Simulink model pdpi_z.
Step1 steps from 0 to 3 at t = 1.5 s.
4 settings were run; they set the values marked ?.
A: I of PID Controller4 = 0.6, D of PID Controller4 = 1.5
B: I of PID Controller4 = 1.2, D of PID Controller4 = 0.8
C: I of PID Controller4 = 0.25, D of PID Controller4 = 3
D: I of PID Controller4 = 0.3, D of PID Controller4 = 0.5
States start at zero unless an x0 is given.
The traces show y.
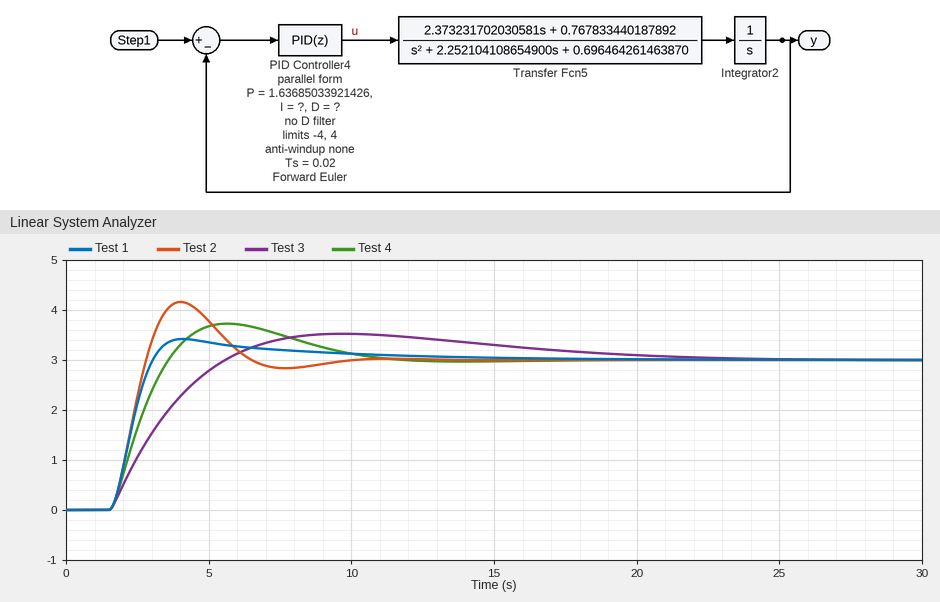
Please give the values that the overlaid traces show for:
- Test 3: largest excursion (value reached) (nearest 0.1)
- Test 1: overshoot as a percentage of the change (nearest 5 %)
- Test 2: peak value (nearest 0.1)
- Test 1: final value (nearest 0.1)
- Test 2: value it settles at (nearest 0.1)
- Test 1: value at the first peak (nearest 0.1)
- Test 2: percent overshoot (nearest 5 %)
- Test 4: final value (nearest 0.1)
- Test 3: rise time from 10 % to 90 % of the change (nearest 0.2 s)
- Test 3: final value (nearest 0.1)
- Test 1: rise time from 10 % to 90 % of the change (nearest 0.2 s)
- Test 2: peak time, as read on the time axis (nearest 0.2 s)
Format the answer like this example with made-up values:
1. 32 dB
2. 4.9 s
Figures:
1. 3.5
2. 15 %
3. 4.2
4. 3.0
5. 3.0
6. 3.4
7. 40 %
8. 3.0
9. 3.0 s
10. 3.0
11. 1.0 s
12. 4.0 s
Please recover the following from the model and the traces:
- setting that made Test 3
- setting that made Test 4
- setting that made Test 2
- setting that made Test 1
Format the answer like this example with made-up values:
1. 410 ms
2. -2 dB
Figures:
1. C
2. A
3. B
4. D
